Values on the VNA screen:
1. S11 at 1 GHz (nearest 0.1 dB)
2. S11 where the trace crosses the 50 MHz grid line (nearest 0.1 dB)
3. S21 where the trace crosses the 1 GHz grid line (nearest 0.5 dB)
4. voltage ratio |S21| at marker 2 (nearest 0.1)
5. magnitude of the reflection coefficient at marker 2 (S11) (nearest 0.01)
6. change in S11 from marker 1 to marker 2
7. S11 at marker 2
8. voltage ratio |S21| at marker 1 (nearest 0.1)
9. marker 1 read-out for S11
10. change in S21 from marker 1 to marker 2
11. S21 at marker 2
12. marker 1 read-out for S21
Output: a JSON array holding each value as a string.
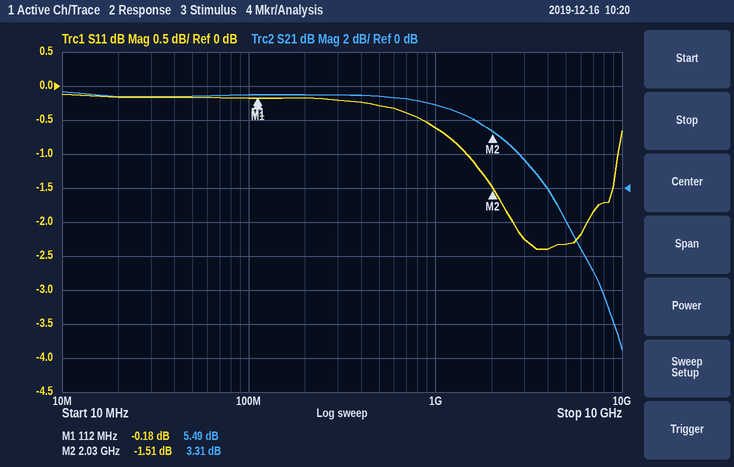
["-0.6 dB", "-0.2 dB", "5.0 dB", "1.5", "0.84", "-1.33 dB", "-1.51 dB", "1.9", "-0.18 dB", "-2.18 dB", "3.31 dB", "5.49 dB"]
